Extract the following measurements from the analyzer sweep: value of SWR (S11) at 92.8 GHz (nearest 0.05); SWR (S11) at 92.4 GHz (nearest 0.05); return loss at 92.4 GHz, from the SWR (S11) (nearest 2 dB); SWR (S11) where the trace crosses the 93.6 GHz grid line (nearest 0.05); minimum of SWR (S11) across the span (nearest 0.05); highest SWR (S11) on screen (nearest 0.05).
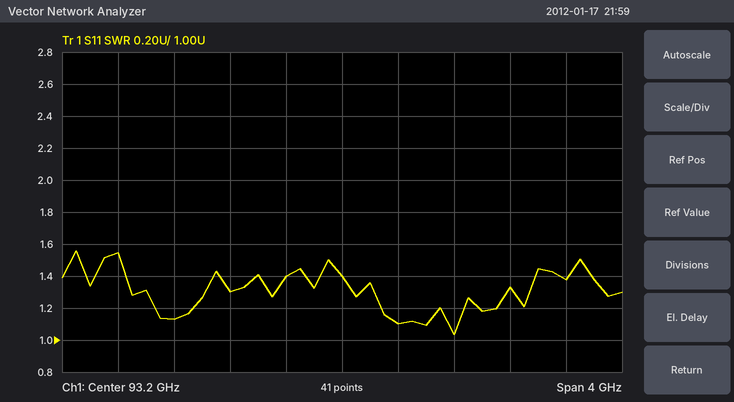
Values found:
1.40
1.30
18 dB
1.10
1.05
1.55
